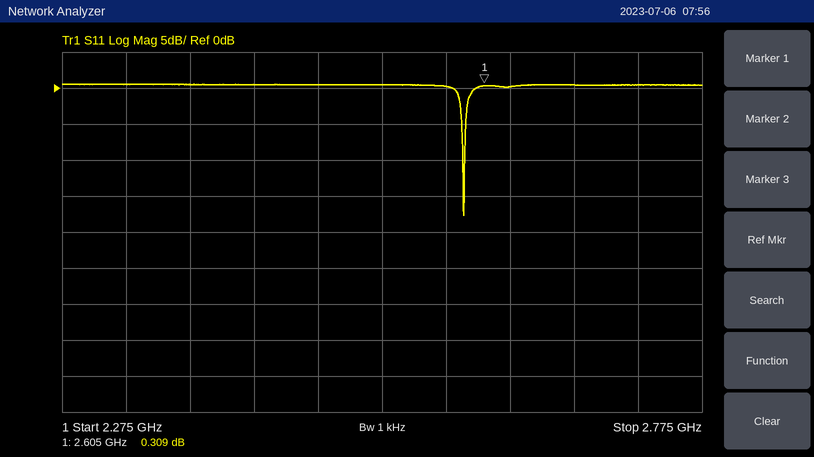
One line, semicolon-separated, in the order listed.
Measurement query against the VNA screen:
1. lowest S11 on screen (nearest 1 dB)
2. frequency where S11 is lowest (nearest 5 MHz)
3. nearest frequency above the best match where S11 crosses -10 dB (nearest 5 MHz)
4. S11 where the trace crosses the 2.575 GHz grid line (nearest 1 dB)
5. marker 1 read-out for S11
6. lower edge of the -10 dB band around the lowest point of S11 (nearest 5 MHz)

-18 dB; 2.590 GHz; 2.590 GHz; 0 dB; 0.309 dB; 2.590 GHz
